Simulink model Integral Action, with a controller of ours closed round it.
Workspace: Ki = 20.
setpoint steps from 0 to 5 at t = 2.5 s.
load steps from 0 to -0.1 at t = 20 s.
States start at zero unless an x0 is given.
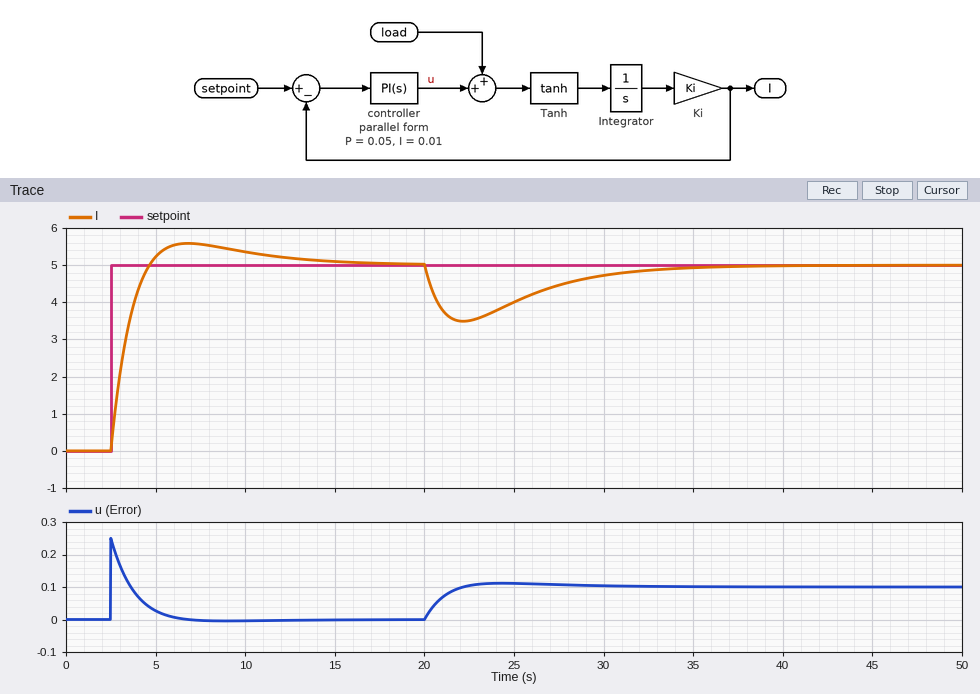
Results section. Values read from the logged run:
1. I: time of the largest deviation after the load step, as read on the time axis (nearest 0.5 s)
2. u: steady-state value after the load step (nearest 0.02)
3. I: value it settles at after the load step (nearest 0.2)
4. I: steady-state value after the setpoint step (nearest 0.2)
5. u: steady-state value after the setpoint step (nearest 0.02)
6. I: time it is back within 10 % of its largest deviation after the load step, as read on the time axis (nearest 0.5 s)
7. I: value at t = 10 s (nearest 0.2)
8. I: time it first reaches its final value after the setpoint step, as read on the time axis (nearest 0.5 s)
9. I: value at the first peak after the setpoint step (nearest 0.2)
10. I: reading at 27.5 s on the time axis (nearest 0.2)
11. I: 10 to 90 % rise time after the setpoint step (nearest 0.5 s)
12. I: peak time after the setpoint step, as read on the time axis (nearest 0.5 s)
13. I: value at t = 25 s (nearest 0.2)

22.0 s
0.10
5.0
5.0
0.00
32.0 s
5.4
4.5 s
5.6
4.4
1.5 s
7.0 s
4.0
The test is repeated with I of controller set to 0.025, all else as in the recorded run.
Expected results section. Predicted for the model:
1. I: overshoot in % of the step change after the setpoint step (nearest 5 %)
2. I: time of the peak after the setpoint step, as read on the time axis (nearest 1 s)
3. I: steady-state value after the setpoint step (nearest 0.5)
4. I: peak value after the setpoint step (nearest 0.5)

20 %
6 s
5.0
6.0
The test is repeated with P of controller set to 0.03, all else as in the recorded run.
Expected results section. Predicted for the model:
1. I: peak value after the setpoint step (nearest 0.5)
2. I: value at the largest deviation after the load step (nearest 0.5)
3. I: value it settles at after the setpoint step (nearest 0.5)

6.0
3.0
5.0
